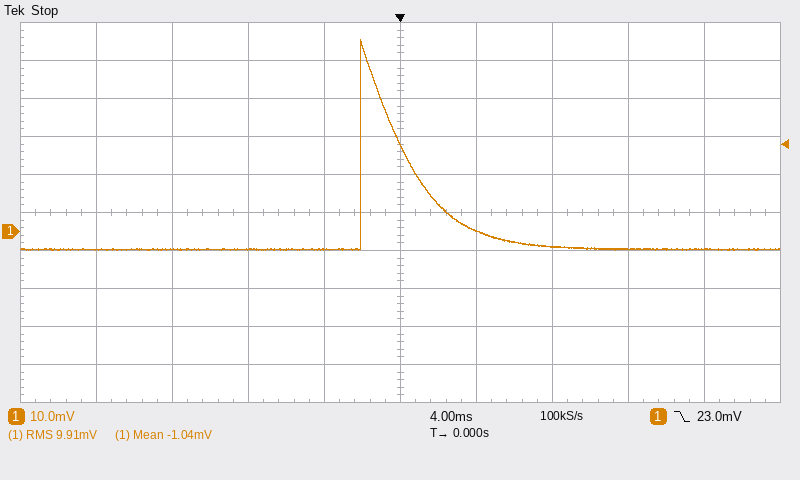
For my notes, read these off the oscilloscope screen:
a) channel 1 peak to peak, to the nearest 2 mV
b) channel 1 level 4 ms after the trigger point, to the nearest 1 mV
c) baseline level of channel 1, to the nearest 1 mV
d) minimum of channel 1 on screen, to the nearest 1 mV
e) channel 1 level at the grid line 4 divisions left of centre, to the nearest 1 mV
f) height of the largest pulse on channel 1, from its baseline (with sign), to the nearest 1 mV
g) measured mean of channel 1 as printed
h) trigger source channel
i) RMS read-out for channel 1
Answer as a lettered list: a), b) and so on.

a) 56 mV
b) 0 mV
c) -5 mV
d) -5 mV
e) -5 mV
f) +55 mV
g) -1.04 mV
h) channel 1
i) 9.91 mV
